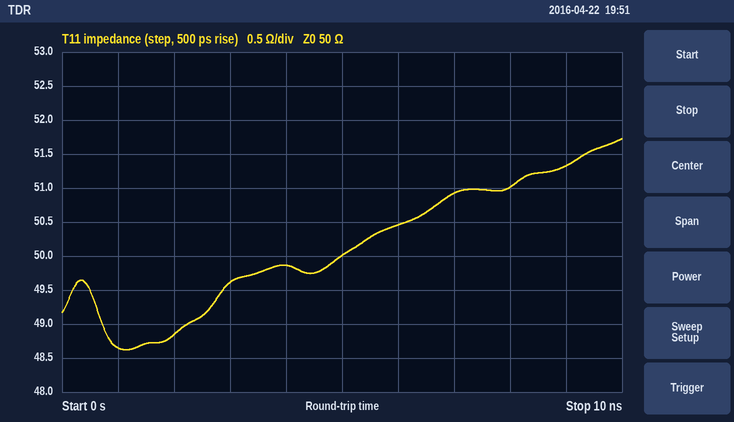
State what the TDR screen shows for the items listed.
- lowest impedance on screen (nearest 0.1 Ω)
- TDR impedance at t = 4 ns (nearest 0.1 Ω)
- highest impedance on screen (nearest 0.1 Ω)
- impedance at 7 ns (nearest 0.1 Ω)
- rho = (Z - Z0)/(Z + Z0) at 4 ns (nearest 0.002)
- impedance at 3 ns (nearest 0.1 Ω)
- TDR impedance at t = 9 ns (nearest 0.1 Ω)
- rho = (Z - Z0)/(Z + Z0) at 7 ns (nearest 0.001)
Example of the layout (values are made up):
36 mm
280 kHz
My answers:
48.6 Ω
49.9 Ω
51.7 Ω
50.9 Ω
-0.002
49.6 Ω
51.3 Ω
+0.009
